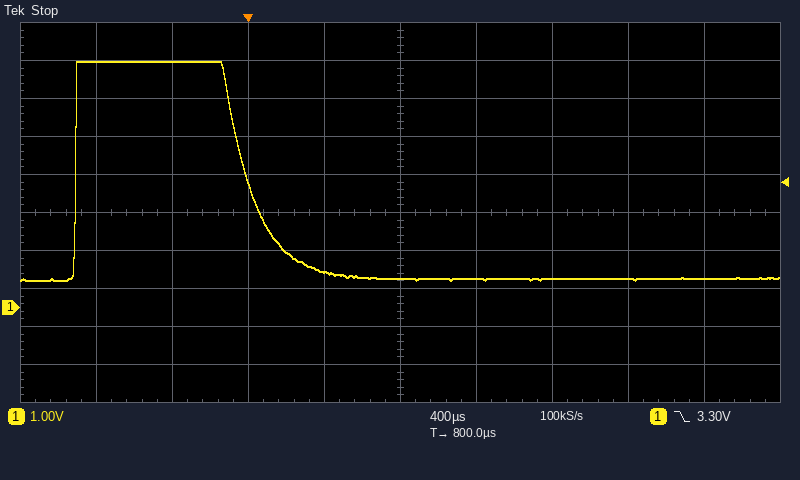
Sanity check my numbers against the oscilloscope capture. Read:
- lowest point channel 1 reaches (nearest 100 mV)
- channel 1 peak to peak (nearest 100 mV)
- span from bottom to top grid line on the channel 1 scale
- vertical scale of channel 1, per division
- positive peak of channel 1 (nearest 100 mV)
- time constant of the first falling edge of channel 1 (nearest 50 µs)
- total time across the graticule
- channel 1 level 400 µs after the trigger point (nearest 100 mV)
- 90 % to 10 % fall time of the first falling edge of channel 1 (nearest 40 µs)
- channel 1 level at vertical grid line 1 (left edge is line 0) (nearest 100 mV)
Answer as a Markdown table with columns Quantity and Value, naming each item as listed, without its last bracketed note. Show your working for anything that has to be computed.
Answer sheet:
| Quantity | Value |
|---|---|
| lowest point channel 1 reaches | 700 mV |
| channel 1 peak to peak | 6.5 V − (700 mV) = 5.8 V |
| span from bottom to top grid line on the channel 1 scale | 10 V |
| vertical scale of channel 1, per division | 1 V |
| positive peak of channel 1 | 6.5 V |
| time constant of the first falling edge of channel 1 | 360 µs / 2.2 ≈ 164 µs, so 150 µs to the nearest 50 µs |
| total time across the graticule | 4 ms |
| channel 1 level 400 µs after the trigger point | 900 mV |
| 90 % to 10 % fall time of the first falling edge of channel 1 | 360 µs |
| channel 1 level at vertical grid line 1 (left edge is line 0) | 6.5 V |
